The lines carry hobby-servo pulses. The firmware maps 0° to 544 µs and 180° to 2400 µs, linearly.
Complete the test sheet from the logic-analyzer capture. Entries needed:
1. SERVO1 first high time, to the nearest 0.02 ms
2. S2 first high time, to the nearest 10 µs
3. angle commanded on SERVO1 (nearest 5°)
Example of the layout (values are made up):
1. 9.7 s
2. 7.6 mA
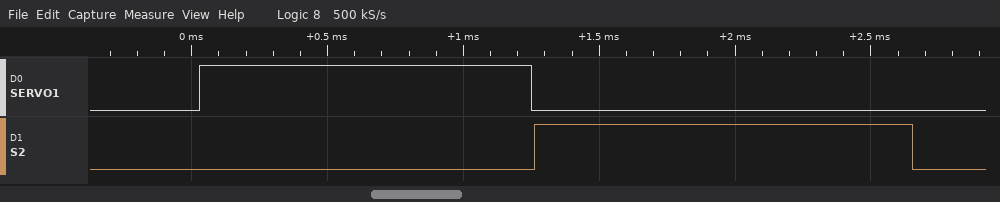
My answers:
1. 1.22 ms
2. 1390 µs
3. 65°
